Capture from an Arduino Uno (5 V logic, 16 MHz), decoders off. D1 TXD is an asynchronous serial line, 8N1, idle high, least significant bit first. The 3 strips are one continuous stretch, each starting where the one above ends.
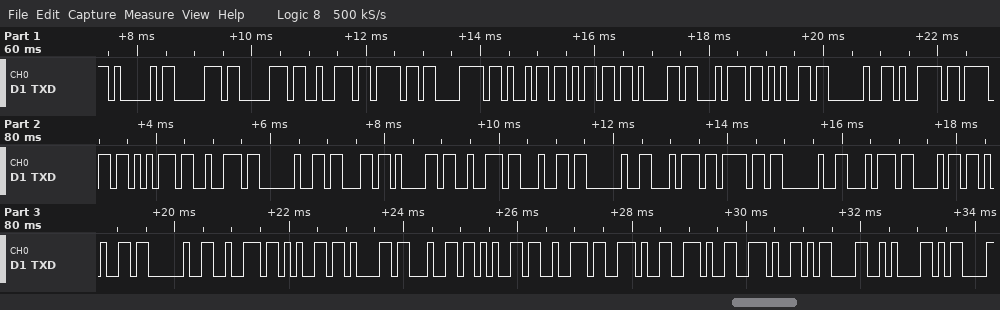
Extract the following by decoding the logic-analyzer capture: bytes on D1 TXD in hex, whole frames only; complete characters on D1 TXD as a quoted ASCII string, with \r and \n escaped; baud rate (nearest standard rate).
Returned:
0x41 0x70 0x70 0x72 0x6F 0x78 0x69 0x6D 0x61 0x74 0x65 0x20 0x79 0x6F 0x75 0x72 0x20 0x63 0x61 0x72 0x64 0x20 0x74 0x6F 0x20 0x74 0x68 0x65 0x20 0x72 0x65 0x61 0x64 0x65 0x72 0x2E 0x2E 0x2E 0x0D 0x0A 0x0D
"Approximate your card to the reader...\r\n\r"
9600 baud
